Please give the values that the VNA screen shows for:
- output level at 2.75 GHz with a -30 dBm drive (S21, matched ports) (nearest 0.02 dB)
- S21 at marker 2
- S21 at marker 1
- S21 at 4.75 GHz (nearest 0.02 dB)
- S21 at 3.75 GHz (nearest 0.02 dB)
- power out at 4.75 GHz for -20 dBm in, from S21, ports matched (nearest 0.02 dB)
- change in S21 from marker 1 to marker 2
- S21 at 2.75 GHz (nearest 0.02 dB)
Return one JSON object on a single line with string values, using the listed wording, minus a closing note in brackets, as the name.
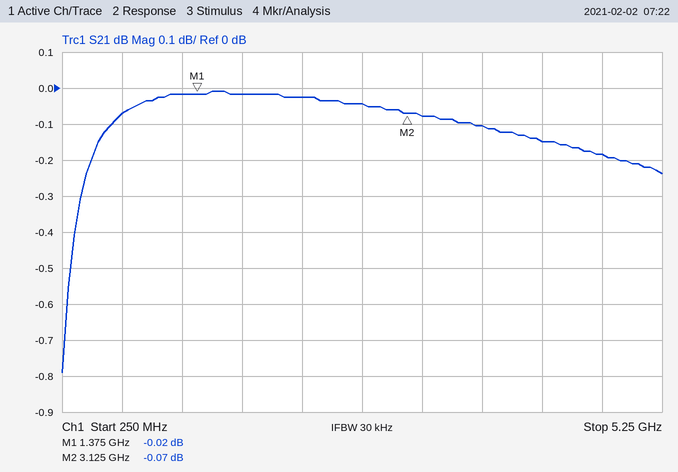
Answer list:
{"output level at 2.75 GHz with a -30 dBm drive (S21, matched ports)": "-30.04 dBm", "S21 at marker 2": "-0.07 dB", "S21 at marker 1": "-0.02 dB", "S21 at 4.75 GHz": "-0.18 dB", "S21 at 3.75 GHz": "-0.10 dB", "power out at 4.75 GHz for -20 dBm in, from S21, ports matched": "-20.18 dBm", "change in S21 from marker 1 to marker 2": "-0.05 dB", "S21 at 2.75 GHz": "-0.04 dB"}
